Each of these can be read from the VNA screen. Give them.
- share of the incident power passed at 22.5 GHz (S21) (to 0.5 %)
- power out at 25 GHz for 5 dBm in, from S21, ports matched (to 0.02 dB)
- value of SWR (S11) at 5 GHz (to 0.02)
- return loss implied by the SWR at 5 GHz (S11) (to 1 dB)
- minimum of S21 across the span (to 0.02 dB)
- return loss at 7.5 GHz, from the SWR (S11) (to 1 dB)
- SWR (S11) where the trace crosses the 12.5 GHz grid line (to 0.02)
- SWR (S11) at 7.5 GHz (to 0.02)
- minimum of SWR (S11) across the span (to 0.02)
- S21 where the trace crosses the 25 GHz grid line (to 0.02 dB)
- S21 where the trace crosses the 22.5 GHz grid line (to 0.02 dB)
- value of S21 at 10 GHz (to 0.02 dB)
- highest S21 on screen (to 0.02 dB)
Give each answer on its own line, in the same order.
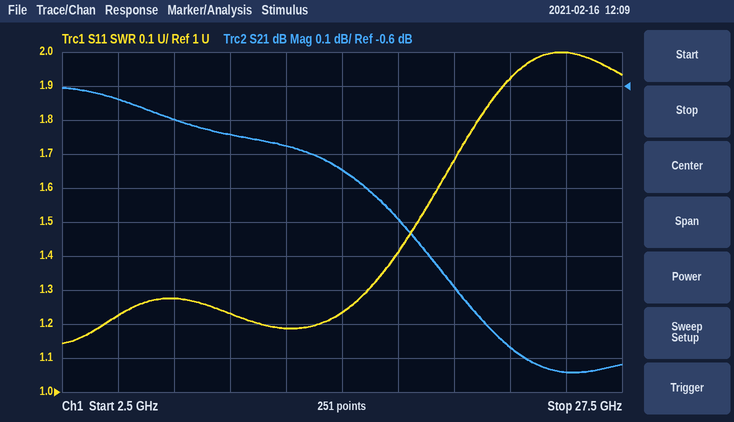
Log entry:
73.0 %
3.56 dBm
1.22
20 dB
-1.44 dB
18 dB
1.18
1.28
1.14
-1.44 dB
-1.36 dB
-0.74 dB
-0.60 dB
